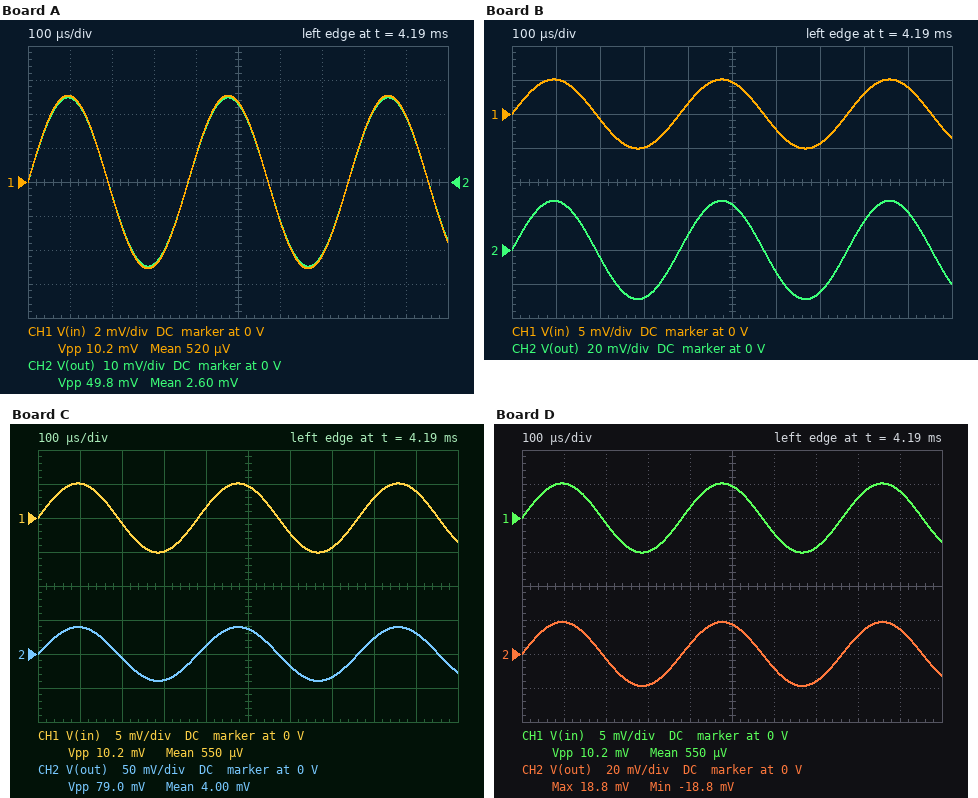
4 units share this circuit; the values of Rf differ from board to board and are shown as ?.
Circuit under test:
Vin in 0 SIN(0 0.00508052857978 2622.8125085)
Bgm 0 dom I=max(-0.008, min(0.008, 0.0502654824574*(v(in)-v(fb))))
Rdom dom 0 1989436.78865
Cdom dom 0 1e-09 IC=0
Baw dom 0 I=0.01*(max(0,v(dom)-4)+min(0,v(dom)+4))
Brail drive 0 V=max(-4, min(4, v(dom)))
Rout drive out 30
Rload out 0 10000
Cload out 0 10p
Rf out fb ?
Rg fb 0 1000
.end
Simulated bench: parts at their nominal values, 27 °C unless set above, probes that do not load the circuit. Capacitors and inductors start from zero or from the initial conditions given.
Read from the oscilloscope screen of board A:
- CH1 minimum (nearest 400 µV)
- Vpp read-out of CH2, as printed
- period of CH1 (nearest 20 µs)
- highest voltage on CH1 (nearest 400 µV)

-5.2 mV
49.8 mV
380 µs
5.2 mV
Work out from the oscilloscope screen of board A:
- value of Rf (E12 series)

3.9 kΩ
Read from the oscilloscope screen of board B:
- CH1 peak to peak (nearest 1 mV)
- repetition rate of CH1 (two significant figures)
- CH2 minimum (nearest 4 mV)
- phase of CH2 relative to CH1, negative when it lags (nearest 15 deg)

10 mV
2.6 kHz
-28 mV
0 deg
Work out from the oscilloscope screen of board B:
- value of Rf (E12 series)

4.7 kΩ
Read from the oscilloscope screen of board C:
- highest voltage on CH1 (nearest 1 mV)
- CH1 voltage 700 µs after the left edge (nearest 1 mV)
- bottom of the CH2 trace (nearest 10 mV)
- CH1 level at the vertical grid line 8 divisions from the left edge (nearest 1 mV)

5 mV
-4 mV
-40 mV
3 mV
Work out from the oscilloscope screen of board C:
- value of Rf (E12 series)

6.8 kΩ
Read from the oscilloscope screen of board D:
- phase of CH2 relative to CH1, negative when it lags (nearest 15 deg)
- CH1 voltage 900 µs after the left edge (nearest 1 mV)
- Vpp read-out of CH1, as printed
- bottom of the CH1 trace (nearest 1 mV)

0 deg
4 mV
10.2 mV
-5 mV
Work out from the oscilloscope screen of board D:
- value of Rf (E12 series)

2.7 kΩ
